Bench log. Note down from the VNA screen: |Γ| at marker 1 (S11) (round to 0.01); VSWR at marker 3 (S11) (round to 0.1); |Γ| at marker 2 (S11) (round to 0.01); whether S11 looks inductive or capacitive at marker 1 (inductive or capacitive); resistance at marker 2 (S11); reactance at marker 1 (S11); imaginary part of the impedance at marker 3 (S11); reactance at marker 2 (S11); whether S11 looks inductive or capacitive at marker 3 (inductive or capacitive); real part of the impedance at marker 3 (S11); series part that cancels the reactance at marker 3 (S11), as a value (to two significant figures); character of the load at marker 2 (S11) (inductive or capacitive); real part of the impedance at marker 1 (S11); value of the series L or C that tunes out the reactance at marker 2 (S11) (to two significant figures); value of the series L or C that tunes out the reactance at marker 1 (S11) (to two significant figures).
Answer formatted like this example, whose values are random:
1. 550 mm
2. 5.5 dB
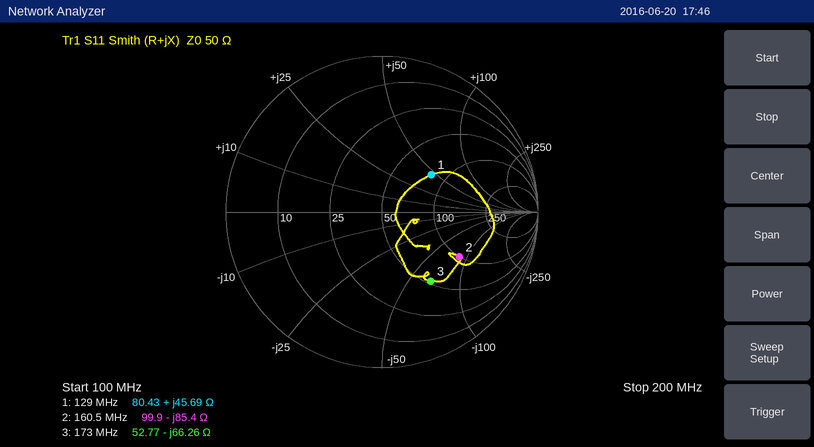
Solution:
1. 0.40
2. 3.4
3. 0.57
4. inductive
5. 99.9 Ω
6. +45.69 Ω
7. -66.26 Ω
8. -85.4 Ω
9. capacitive
10. 52.77 Ω
11. 61 nH
12. capacitive
13. 80.43 Ω
14. 85 nH
15. 27 pF
